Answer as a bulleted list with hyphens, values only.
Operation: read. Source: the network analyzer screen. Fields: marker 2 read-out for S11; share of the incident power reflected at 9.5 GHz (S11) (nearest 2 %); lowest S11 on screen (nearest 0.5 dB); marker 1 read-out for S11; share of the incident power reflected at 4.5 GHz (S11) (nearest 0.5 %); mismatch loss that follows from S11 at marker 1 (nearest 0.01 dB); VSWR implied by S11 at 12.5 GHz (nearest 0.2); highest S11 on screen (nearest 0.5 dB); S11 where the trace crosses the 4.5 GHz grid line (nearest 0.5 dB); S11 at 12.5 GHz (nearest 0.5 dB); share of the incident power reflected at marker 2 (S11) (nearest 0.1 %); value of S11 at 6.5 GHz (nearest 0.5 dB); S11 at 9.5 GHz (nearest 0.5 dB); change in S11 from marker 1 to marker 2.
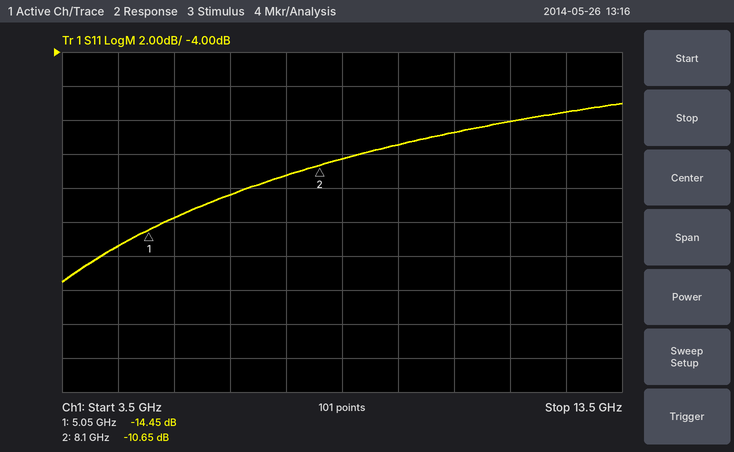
- -10.65 dB
- 12 %
- -17.5 dB
- -14.45 dB
- 3.0 %
- 0.16 dB
- 2.4
- -7.0 dB
- -15.5 dB
- -7.5 dB
- 8.6 %
- -12.5 dB
- -9.5 dB
- 3.80 dB
